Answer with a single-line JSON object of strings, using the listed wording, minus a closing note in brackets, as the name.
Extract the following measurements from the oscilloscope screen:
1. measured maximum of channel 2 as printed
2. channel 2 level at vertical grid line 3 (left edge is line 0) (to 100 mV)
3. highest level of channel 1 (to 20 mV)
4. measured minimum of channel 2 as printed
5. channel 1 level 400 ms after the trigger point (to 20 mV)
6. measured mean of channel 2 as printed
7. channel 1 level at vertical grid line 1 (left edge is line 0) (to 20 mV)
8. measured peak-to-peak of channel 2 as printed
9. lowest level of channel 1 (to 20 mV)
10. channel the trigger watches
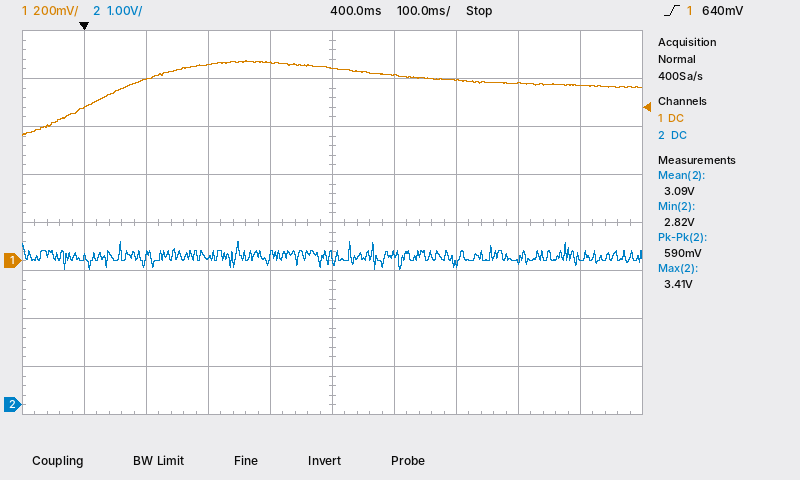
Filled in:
{"measured maximum of channel 2 as printed": "3.41 V", "channel 2 level at vertical grid line 3 (left edge is line 0)": "3.1 V", "highest level of channel 1": "840 mV", "measured minimum of channel 2 as printed": "2.82 V", "channel 1 level 400 ms after the trigger point": "800 mV", "measured mean of channel 2 as printed": "3.09 V", "channel 1 level at vertical grid line 1 (left edge is line 0)": "640 mV", "measured peak-to-peak of channel 2 as printed": "590 mV", "lowest level of channel 1": "520 mV", "channel the trigger watches": "channel 1"}
